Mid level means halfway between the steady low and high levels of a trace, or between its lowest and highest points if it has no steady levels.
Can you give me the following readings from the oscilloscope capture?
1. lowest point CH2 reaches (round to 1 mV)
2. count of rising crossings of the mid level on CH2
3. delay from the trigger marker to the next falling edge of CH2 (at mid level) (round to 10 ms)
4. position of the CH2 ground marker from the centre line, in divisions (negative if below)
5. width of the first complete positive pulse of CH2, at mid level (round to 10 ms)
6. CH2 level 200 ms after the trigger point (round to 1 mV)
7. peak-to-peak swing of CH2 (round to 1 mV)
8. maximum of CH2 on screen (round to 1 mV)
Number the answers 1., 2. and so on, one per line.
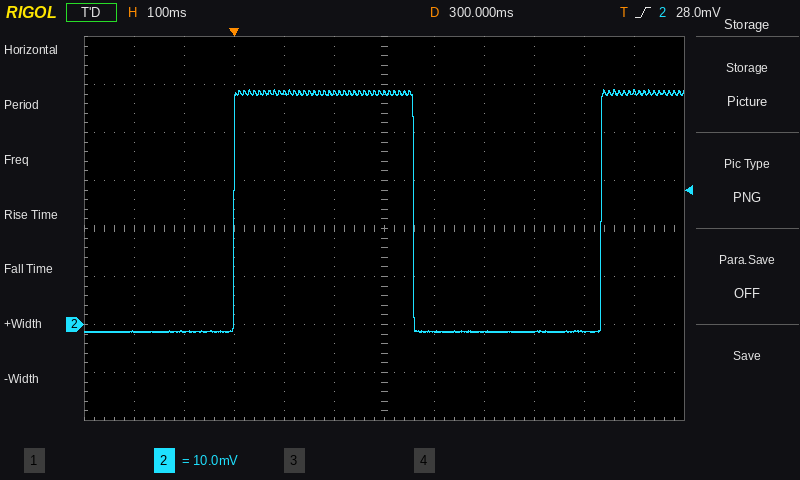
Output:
1. -2 mV
2. 2
3. 360 ms
4. -2.0 div
5. 360 ms
6. 48 mV
7. 51 mV
8. 49 mV
